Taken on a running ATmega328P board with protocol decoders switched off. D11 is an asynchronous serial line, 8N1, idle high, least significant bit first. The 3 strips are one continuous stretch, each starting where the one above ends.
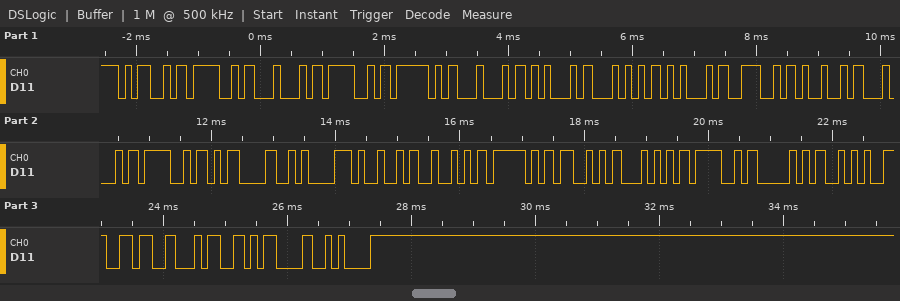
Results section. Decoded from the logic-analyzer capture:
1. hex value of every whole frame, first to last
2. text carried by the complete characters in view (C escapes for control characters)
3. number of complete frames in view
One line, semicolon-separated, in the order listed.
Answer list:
0x4D 0x4F 0x44 0x4F 0x5F 0x44 0x45 0x54 0x45 0x4E 0x49 0x44 0x4F 0x0D 0x0A 0x49 0x52 0x5F 0x53 0x54 0x4F 0x50 0x2A 0x36 0x34 0x0D 0x0A; "MODO_DETENIDO\r\nIR_STOP*64\r\n"; 27
